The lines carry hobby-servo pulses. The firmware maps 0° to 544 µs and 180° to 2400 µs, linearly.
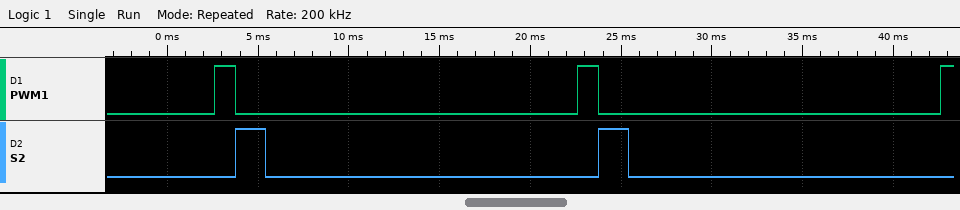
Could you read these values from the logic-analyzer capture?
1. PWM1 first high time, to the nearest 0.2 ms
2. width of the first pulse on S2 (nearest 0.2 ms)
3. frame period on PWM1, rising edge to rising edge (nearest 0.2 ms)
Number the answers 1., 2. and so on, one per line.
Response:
1. 1.2 ms
2. 1.6 ms
3. 20.0 ms
